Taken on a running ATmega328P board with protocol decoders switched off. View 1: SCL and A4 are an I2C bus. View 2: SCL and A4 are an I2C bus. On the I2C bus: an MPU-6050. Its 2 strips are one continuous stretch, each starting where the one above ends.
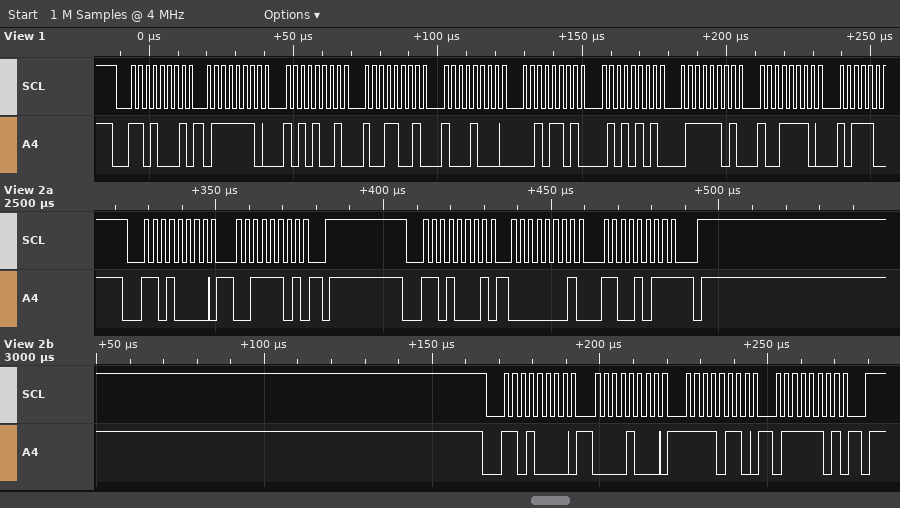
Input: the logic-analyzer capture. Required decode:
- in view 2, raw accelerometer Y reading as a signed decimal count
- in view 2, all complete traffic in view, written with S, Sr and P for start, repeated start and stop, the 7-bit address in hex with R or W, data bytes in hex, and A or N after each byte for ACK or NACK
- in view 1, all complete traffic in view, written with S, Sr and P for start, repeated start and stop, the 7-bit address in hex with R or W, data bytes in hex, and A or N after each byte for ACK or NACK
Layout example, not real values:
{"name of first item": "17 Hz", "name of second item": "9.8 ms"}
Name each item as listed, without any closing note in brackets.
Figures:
{"in view 2, raw accelerometer Y reading as a signed decimal count": "459", "in view 2, all complete traffic in view, written with S, Sr and P for start, repeated start and stop, the 7-bit address in hex with R or W, data bytes in hex, and A or N after each byte for ACK or NACK": "S 68W A 3D A P S 68R A 01 A CB N P S 68W A 08 A F6 A 7D A P", "in view 1, all complete traffic in view, written with S, Sr and P for start, repeated start and stop, the 7-bit address in hex with R or W, data bytes in hex, and A or N after each byte for ACK or NACK": "S 68R A 7E A A9 A 99 A 88 A 2D A 55 A 7D A 9E A"}
